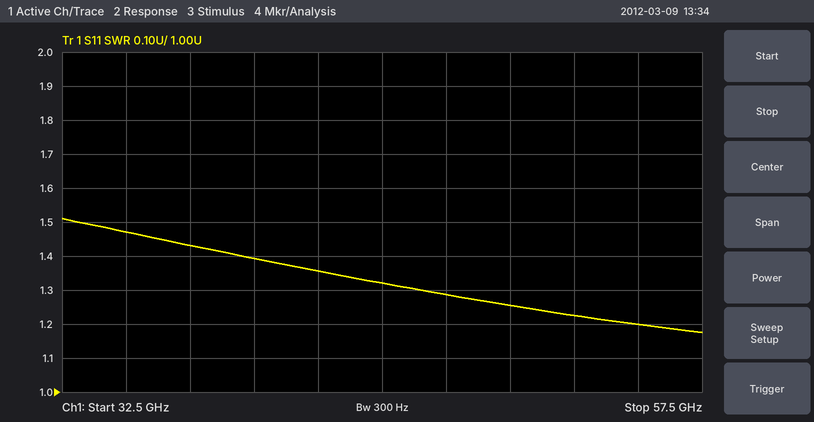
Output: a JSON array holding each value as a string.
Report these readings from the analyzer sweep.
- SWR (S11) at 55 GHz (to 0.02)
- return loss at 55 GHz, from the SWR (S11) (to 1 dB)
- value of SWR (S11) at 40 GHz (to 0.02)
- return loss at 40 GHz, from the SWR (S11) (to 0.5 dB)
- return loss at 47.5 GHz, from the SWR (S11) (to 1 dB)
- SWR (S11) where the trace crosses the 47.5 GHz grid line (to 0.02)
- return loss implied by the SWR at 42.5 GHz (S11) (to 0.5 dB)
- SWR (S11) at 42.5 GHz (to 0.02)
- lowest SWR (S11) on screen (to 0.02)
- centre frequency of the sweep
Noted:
["1.20", "21 dB", "1.40", "15.5 dB", "18 dB", "1.28", "16.5 dB", "1.36", "1.18", "45 GHz"]
